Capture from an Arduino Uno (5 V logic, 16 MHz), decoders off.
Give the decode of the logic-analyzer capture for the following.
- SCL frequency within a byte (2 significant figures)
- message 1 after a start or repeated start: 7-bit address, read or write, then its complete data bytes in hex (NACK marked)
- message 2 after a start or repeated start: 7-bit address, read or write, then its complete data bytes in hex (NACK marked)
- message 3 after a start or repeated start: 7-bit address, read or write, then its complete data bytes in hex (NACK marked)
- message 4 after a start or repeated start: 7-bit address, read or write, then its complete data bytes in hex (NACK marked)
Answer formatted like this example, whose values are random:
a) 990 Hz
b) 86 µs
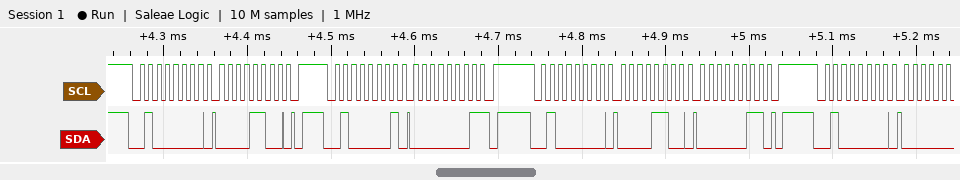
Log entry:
a) 100 kHz
b) 0x20 write: 0C
c) 0x20 read: 01 NACK
d) 0x20 write: 0C 03
e) 0x20 write
